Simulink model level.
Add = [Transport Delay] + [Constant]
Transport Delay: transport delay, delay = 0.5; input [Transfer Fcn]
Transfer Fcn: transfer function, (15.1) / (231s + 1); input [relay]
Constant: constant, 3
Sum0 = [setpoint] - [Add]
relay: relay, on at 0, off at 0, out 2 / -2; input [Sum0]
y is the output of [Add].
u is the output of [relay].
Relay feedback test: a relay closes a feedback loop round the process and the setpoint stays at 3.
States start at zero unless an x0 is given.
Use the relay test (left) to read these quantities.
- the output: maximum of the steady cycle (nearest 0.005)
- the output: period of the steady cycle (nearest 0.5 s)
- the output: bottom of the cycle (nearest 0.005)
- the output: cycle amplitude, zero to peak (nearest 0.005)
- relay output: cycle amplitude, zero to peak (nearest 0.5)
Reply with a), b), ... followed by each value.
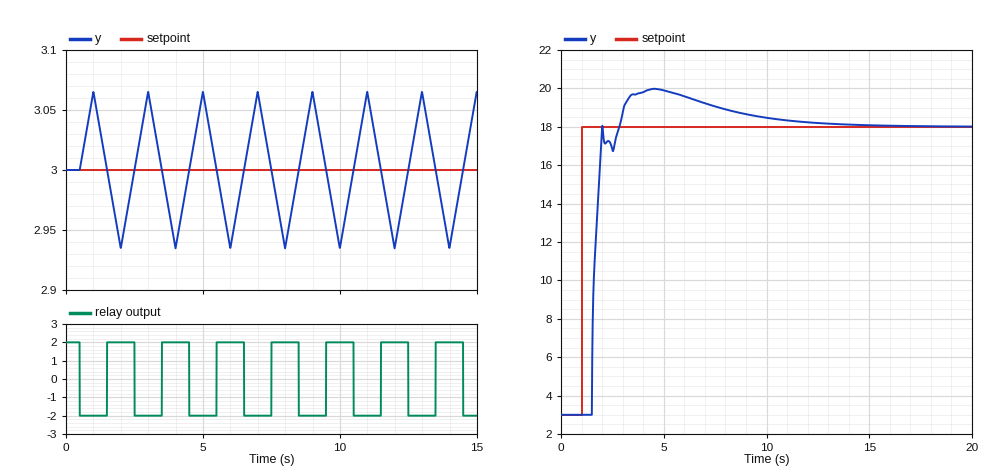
a) 3.065
b) 2.0 s
c) 2.935
d) 0.065
e) 2.0
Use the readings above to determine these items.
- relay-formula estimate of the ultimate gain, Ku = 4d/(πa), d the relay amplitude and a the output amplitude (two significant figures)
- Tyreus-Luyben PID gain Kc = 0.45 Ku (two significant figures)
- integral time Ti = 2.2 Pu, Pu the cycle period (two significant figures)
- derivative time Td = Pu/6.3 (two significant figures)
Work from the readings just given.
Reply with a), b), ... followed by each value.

a) 39
b) 18
c) 4.4 s
d) 0.32 s
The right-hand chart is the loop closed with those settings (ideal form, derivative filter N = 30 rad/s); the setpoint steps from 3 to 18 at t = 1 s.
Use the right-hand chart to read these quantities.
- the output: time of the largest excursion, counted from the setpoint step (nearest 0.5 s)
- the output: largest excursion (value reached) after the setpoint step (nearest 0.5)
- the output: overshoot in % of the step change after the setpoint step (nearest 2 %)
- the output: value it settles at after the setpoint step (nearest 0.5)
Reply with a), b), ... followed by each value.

a) 3.5 s
b) 20.0
c) 14 %
d) 18.0
